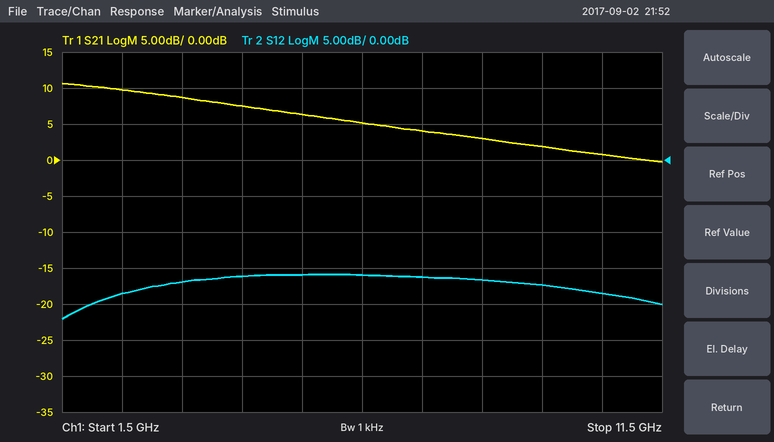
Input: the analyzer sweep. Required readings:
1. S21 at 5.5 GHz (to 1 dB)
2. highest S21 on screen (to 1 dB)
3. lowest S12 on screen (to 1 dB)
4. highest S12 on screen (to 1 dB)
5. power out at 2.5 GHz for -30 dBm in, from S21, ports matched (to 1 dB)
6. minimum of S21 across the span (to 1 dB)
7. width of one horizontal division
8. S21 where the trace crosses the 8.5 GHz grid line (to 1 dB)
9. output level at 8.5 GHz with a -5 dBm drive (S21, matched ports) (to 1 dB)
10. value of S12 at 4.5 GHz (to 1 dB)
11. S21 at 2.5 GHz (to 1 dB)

6 dB
11 dB
-22 dB
-16 dB
-20 dBm
0 dB
1 GHz
3 dB
-2 dBm
-16 dB
10 dB
